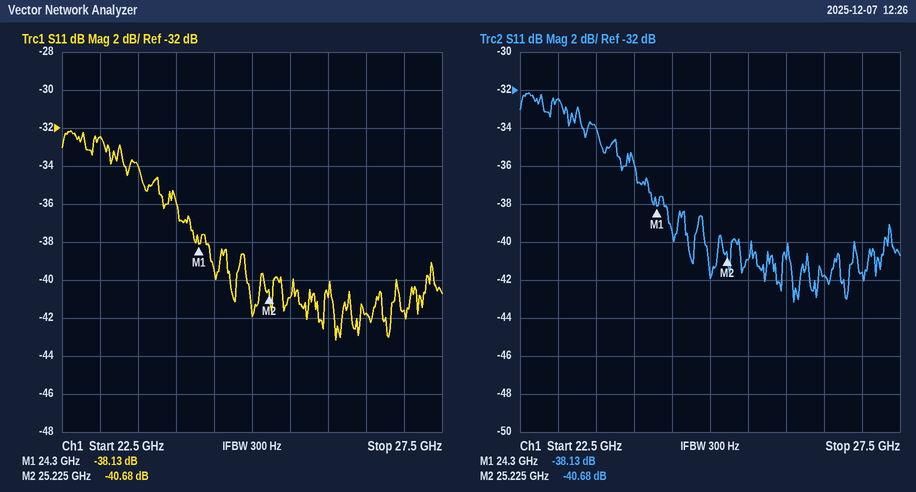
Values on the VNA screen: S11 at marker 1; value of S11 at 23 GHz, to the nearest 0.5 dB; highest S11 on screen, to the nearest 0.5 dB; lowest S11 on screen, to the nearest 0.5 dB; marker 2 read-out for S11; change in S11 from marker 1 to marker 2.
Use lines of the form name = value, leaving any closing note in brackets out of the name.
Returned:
S11 at marker 1 = -38.13 dB
value of S11 at 23 GHz, to the nearest 0.5 dB = -32.5 dB
highest S11 on screen, to the nearest 0.5 dB = -32.0 dB
lowest S11 on screen, to the nearest 0.5 dB = -43.0 dB
marker 2 read-out for S11 = -40.68 dB
change in S11 from marker 1 to marker 2 = -2.55 dB
